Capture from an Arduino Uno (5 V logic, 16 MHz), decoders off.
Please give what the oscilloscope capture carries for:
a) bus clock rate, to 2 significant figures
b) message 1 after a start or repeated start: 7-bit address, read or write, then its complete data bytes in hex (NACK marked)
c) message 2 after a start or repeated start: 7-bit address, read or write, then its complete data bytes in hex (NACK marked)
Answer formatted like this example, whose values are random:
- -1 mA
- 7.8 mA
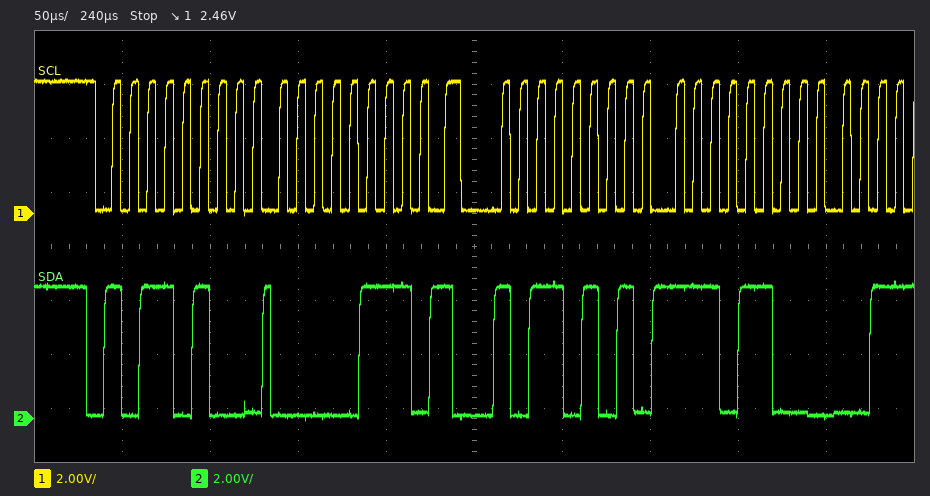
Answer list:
- 100 kHz
- 0x5A write: 07
- 0x5A read: EC
